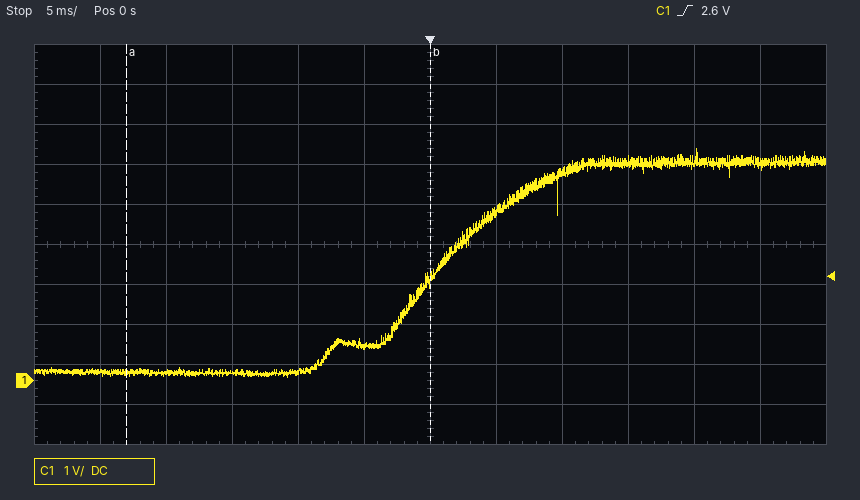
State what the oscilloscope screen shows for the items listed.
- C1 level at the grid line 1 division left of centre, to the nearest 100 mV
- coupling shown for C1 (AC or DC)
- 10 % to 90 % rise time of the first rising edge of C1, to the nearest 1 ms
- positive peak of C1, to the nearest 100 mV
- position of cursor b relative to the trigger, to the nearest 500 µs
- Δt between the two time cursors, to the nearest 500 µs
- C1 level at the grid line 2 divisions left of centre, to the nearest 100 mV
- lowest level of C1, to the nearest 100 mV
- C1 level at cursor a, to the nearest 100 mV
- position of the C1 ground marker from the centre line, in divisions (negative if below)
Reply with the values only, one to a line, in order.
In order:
900 mV
DC
16 ms
5.8 V
0.0 ms
23.0 ms
200 mV
100 mV
200 mV
-3.4 div
